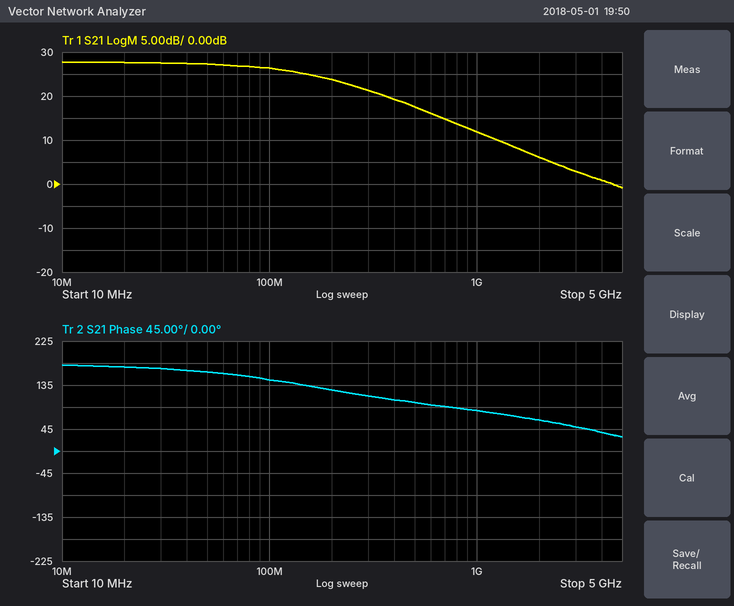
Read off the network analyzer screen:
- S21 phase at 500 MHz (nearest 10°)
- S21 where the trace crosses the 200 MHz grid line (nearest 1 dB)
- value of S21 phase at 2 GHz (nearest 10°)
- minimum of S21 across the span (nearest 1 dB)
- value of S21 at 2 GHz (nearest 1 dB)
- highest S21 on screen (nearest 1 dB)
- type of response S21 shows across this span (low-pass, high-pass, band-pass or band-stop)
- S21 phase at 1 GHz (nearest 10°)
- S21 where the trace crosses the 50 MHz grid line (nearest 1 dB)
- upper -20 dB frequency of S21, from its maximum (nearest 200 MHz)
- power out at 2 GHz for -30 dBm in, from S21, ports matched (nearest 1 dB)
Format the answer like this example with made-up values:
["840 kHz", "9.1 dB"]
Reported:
["100°", "24 dB", "60°", "-1 dB", "6 dB", "28 dB", "low-pass", "80°", "27 dB", "1.6 GHz", "-24 dBm"]
